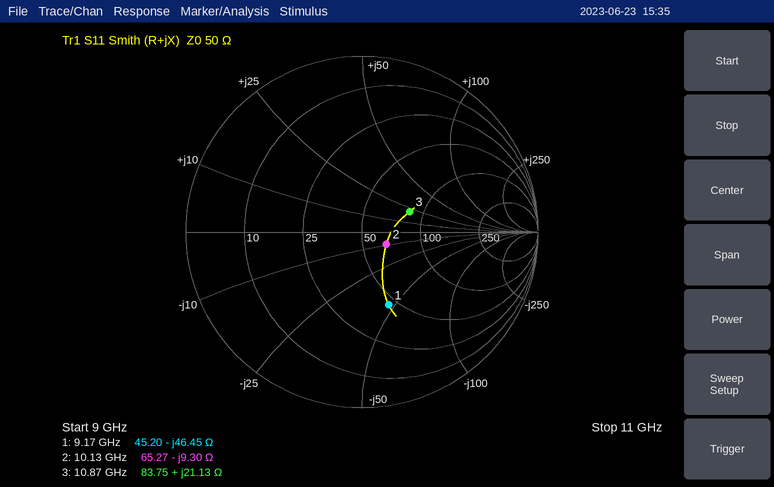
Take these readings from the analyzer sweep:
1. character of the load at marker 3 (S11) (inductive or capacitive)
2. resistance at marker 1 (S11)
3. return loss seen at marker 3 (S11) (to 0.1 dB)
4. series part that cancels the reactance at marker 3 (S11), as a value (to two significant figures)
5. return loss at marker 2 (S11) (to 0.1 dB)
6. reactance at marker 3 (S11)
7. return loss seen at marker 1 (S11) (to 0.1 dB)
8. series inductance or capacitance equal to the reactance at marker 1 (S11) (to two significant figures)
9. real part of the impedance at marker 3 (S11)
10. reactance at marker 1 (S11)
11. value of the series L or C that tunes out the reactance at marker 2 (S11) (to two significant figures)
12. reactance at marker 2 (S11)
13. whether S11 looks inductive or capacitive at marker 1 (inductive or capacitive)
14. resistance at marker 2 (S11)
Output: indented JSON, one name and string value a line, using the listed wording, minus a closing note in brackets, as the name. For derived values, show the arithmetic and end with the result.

{
  "character of the load at marker 3 (S11)": "inductive",
  "resistance at marker 1": "45.20 Ω",
  "return loss seen at marker 3 (S11)": "10.6 dB",
  "series part that cancels the reactance at marker 3 (S11), as a value": "C = 1/(2π × 10.87 GHz × 21.13 Ω) ≈ 693 fF, so 690 fF to two significant figures",
  "return loss at marker 2 (S11)": "16.2 dB",
  "reactance at marker 3": "+21.13 Ω",
  "return loss seen at marker 1 (S11)": "7.1 dB",
  "series inductance or capacitance equal to the reactance at marker 1 (S11)": "C = 1/(2π × 9.17 GHz × 46.45 Ω) ≈ 374 fF, so 370 fF to two significant figures",
  "real part of the impedance at marker 3": "83.75 Ω",
  "reactance at marker 1": "-46.45 Ω",
  "value of the series L or C that tunes out the reactance at marker 2 (S11)": "L = 9.3 Ω/(2π × 10.13 GHz) ≈ 146 pH, so 150 pH to two significant figures",
  "reactance at marker 2": "-9.30 Ω",
  "whether S11 looks inductive or capacitive at marker 1": "capacitive",
  "resistance at marker 2": "65.27 Ω"
}
